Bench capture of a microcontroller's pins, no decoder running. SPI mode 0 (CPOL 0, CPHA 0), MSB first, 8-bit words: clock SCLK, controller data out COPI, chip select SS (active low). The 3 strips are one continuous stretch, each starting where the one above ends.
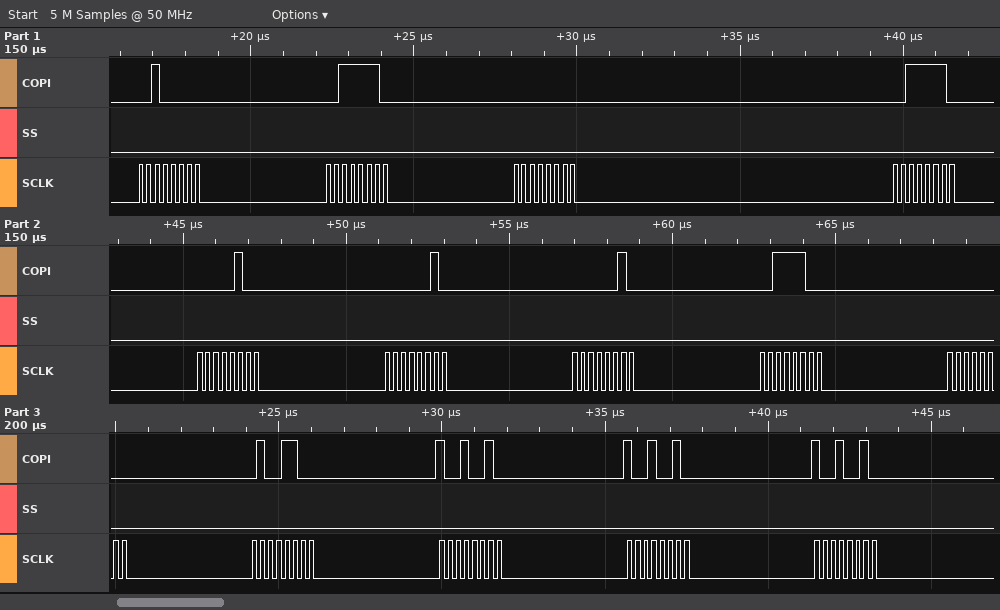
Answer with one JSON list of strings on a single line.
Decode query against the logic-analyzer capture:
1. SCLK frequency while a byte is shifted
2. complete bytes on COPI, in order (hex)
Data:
["4 MHz", "20 3E 00 3E 04 02 02 3C 00 4C 92 92 92"]
